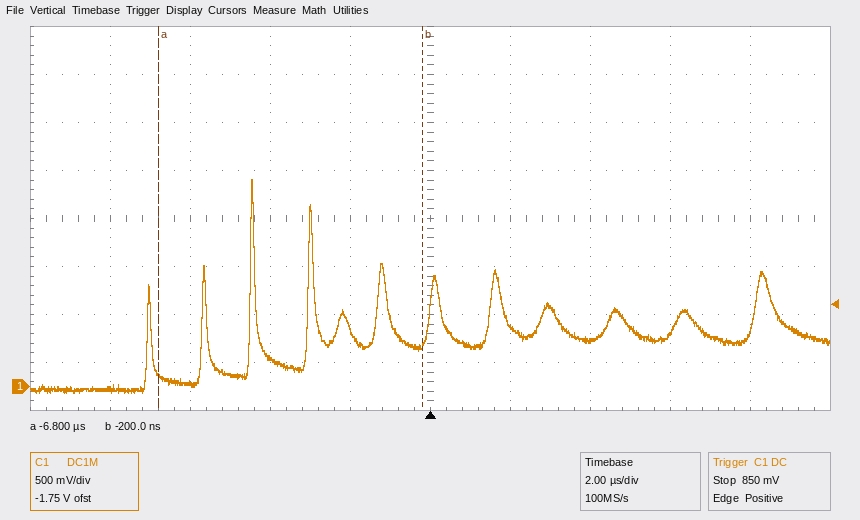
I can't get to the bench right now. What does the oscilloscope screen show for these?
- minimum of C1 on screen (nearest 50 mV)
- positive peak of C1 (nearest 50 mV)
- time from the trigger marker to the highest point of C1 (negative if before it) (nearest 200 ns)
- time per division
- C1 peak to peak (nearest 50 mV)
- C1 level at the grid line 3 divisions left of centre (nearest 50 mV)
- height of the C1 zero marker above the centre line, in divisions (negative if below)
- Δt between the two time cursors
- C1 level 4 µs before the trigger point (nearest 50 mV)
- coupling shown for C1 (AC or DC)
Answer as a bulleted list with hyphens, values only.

- -50 mV
- 2.15 V
- -4.4 µs
- 2 µs
- 2.20 V
- 50 mV
- -3.5 div
- 6.6 µs
- 300 mV
- DC
